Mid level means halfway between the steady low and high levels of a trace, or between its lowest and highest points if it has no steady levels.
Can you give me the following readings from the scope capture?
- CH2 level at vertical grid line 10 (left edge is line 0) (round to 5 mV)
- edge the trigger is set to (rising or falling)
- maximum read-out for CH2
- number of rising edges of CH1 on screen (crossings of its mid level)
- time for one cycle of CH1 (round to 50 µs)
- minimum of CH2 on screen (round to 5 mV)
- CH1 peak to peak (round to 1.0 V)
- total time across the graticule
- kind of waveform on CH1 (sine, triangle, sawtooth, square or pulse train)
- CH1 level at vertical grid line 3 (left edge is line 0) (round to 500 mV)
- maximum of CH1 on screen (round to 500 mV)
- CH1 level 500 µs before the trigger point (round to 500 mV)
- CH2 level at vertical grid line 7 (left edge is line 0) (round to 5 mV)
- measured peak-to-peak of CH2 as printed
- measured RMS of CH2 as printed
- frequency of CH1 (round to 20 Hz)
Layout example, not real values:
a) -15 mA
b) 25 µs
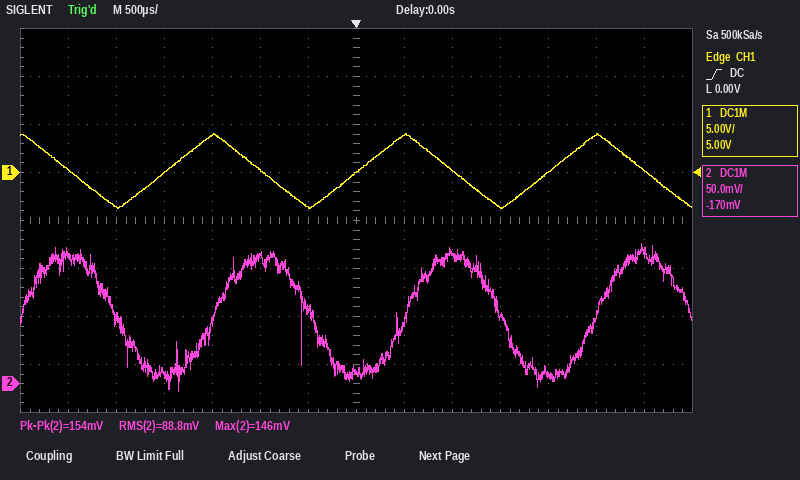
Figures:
a) 70 mV
b) rising
c) 146 mV
d) 3
e) 2.00 ms
f) -10 mV
g) 8.0 V
h) 7 ms
i) triangle
j) 0.0 V
k) 4.0 V
l) -3.5 V
m) 10 mV
n) 154 mV
o) 88.8 mV
p) 500 Hz
